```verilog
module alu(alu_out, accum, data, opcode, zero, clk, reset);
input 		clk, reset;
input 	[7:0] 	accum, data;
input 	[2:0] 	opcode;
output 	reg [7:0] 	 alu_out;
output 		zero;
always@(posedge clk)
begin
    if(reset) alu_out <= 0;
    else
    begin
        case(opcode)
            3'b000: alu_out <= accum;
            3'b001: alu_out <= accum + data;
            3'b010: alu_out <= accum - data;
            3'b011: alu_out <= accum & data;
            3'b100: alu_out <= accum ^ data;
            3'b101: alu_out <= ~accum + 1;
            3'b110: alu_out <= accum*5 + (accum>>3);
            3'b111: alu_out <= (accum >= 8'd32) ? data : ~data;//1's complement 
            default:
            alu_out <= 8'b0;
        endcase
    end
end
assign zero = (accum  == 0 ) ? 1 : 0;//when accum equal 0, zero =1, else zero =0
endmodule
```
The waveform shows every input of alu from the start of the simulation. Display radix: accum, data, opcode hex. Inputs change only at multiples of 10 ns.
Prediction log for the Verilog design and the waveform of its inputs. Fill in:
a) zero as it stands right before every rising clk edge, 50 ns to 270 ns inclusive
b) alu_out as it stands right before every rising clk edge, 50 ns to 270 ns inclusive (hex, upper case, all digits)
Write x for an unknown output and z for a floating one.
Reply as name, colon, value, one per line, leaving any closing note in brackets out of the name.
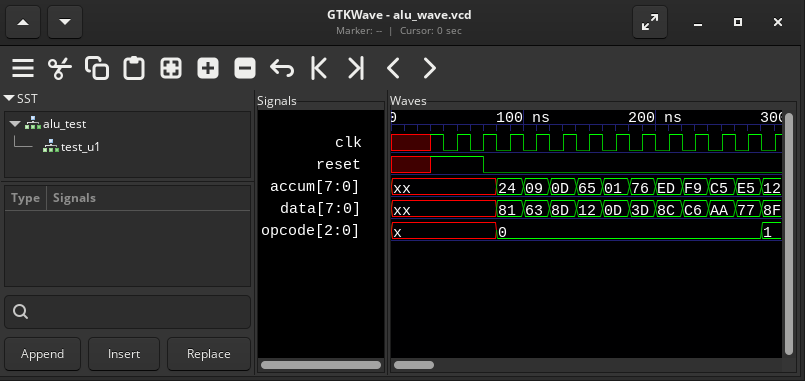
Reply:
zero as it stands right before every rising clk edge, 50 ns to 270 ns inclusive: x x 0 0 0 0 0 0 0 0 0 0
alu_out as it stands right before every rising clk edge, 50 ns to 270 ns inclusive: 00, 00, 00, 24, 09, 0D, 65, 01, 76, ED, F9, C5
